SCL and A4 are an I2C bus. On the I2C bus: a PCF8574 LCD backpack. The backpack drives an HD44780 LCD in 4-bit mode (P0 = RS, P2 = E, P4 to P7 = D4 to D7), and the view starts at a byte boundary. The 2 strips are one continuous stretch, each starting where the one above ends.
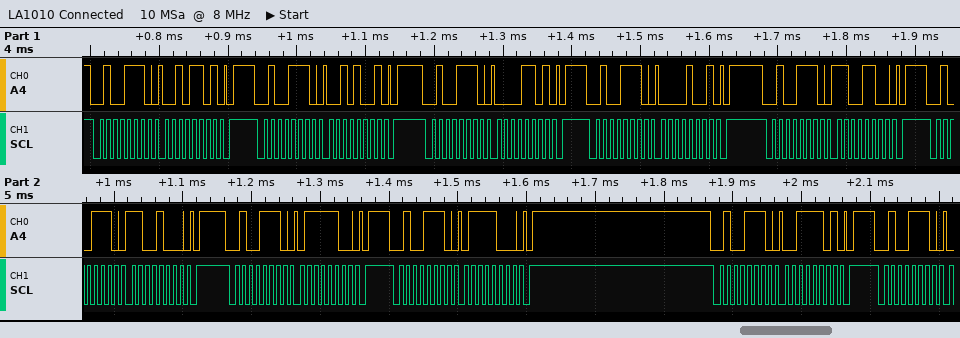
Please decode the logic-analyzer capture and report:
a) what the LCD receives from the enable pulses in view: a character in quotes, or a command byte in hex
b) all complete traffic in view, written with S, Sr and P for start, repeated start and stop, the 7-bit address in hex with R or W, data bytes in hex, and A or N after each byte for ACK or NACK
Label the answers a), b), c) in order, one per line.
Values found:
a) ' ' 0xC7
b) S 27W A 2D A P S 27W A 29 A P S 27W A 0D A P S 27W A 09 A P S 27W A CC A P S 27W A C8 A P S 27W A 7C A P S 27W A 78 A P S 27W A 3D A P S 27W A
